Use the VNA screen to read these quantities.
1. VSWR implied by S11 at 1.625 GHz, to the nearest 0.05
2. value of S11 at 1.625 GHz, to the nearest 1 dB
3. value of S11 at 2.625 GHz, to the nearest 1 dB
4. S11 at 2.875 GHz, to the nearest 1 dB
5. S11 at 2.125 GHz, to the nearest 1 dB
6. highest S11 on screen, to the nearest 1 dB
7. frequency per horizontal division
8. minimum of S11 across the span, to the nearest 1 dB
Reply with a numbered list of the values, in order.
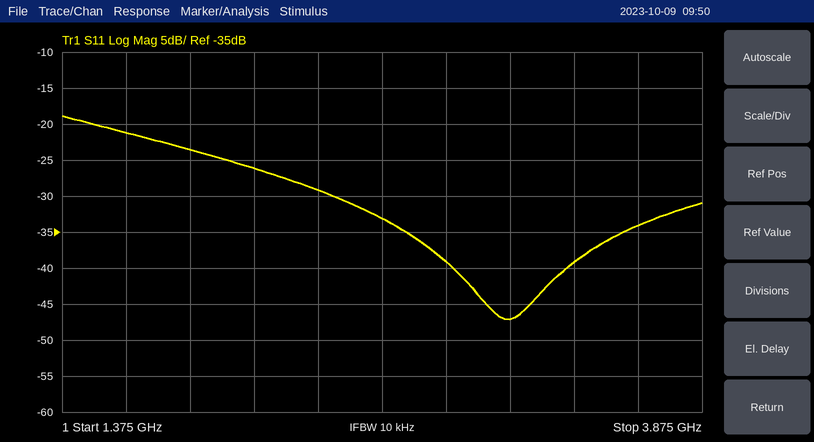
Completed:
1. 1.20
2. -21 dB
3. -33 dB
4. -39 dB
5. -26 dB
6. -19 dB
7. 250 MHz
8. -47 dB
